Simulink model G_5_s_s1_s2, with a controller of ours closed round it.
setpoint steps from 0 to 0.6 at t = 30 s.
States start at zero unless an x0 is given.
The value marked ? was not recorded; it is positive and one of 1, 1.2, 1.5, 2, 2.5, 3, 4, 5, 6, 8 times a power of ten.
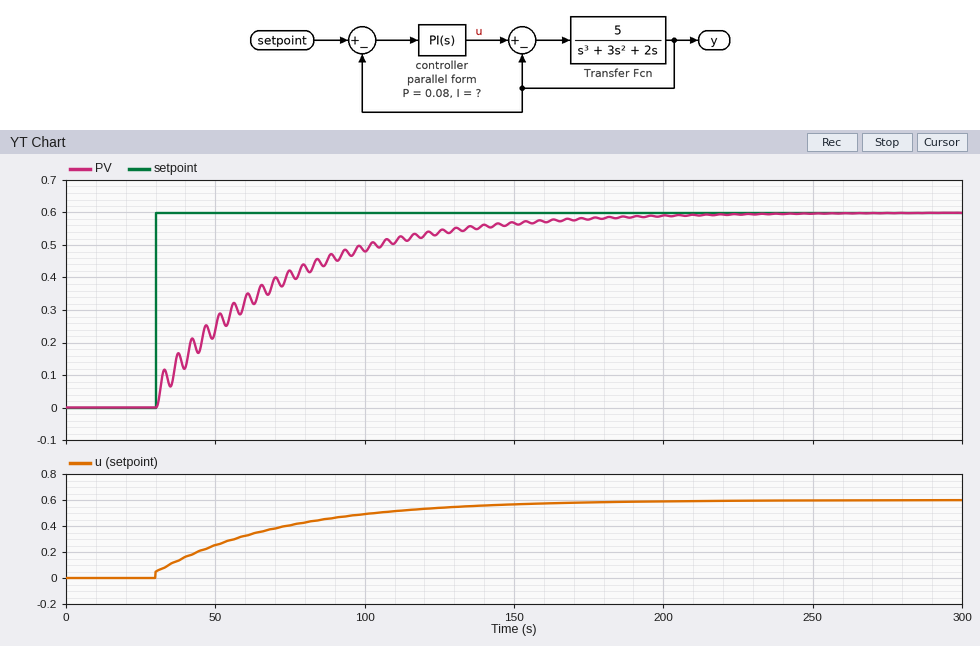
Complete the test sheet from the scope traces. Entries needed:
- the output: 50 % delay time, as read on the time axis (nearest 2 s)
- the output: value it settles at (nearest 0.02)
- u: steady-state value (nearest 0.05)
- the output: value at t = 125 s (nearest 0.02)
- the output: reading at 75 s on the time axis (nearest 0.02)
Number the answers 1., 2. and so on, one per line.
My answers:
1. 56 s
2. 0.60
3. 0.60
4. 0.54
5. 0.42
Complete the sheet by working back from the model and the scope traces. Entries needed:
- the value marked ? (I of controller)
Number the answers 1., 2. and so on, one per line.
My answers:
1. 0.025
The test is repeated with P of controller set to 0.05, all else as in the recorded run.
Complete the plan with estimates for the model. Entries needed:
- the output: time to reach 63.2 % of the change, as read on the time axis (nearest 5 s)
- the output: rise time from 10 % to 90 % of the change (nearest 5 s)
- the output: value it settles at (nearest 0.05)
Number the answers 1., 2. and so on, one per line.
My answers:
1. 70 s
2. 90 s
3. 0.60
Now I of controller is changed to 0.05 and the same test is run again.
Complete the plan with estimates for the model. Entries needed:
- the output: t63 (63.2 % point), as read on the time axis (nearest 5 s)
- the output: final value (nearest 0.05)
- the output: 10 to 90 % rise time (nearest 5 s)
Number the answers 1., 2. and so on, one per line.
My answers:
1. 45 s
2. 0.60
3. 40 s
